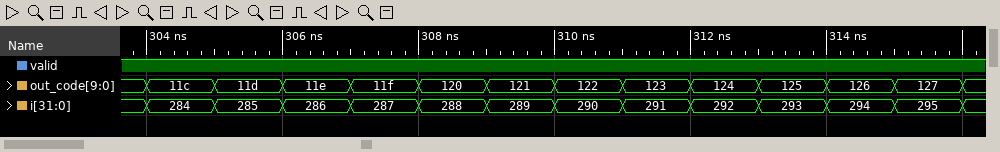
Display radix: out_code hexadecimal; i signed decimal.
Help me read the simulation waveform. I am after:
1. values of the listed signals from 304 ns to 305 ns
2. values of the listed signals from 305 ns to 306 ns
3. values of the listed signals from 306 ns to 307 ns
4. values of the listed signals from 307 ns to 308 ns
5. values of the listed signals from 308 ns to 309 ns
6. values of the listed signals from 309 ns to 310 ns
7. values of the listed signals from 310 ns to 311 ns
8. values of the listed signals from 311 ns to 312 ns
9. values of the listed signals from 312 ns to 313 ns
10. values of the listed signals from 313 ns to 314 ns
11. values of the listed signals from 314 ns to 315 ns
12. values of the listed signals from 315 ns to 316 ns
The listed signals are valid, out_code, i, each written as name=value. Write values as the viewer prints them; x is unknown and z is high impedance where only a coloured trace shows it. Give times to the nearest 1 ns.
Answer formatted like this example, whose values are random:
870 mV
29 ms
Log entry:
valid=1, out_code=11c, i=284
valid=1, out_code=11d, i=285
valid=1, out_code=11e, i=286
valid=1, out_code=11f, i=287
valid=1, out_code=120, i=288
valid=1, out_code=121, i=289
valid=1, out_code=122, i=290
valid=1, out_code=123, i=291
valid=1, out_code=124, i=292
valid=1, out_code=125, i=293
valid=1, out_code=126, i=294
valid=1, out_code=127, i=295
